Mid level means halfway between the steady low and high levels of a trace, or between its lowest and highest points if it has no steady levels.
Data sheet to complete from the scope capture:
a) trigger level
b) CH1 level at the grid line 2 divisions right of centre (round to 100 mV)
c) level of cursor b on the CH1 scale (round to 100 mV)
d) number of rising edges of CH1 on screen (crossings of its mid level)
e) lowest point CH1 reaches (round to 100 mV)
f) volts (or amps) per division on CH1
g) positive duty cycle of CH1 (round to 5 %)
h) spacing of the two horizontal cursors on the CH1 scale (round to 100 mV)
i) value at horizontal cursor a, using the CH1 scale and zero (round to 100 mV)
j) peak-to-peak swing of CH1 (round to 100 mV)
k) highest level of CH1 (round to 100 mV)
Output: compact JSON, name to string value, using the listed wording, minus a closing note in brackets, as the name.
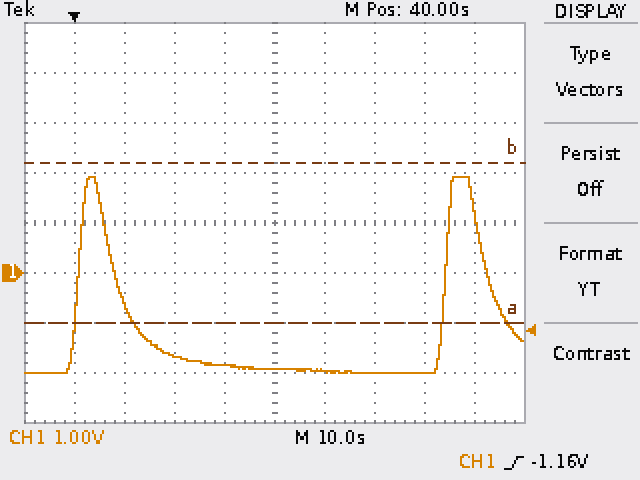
{"trigger level": "-1.16 V", "CH1 level at the grid line 2 divisions right of centre": "-2.0 V", "level of cursor b on the CH1 scale": "2.2 V", "number of rising edges of CH1 on screen": "2", "lowest point CH1 reaches": "-2.0 V", "volts (or amps) per division on CH1": "1 V", "positive duty cycle of CH1": "10 %", "spacing of the two horizontal cursors on the CH1 scale": "3.2 V", "value at horizontal cursor a, using the CH1 scale and zero": "-1.0 V", "peak-to-peak swing of CH1": "3.9 V", "highest level of CH1": "1.9 V"}
